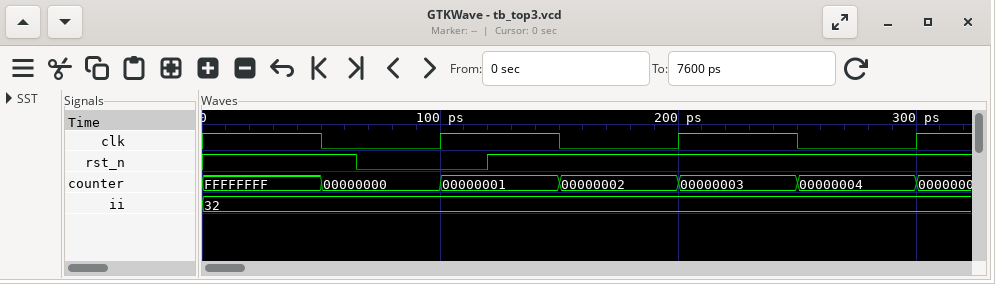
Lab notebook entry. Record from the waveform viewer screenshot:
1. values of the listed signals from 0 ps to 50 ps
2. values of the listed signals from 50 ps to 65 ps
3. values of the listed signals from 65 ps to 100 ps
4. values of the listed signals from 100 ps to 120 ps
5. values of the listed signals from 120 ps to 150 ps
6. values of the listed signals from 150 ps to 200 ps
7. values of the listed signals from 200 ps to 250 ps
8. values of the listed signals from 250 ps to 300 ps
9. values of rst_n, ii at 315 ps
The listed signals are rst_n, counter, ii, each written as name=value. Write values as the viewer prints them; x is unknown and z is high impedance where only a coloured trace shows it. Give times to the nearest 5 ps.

rst_n=1, counter=FFFFFFFF, ii=32
rst_n=1, counter=00000000, ii=32
rst_n=0, counter=00000000, ii=32
rst_n=0, counter=00000001, ii=32
rst_n=1, counter=00000001, ii=32
rst_n=1, counter=00000002, ii=32
rst_n=1, counter=00000003, ii=32
rst_n=1, counter=00000004, ii=32
rst_n=1, ii=32
